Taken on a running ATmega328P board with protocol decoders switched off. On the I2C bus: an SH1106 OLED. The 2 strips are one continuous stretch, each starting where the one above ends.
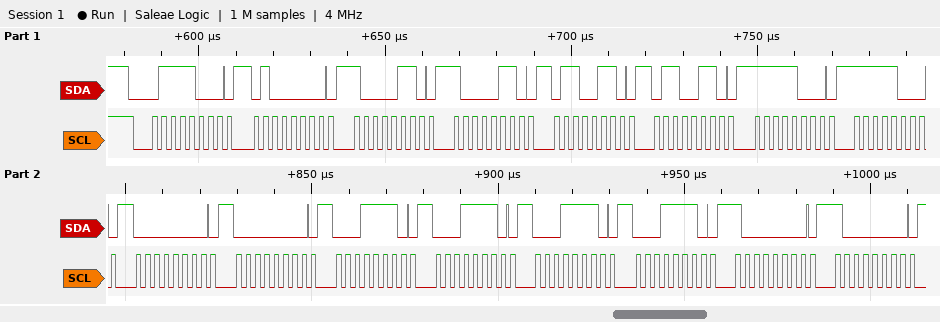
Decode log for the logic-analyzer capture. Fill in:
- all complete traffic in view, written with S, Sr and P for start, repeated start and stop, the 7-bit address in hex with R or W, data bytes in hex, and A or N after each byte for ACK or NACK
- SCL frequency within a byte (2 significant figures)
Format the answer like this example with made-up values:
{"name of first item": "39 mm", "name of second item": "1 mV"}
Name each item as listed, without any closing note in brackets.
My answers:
{"all complete traffic in view, written with S, Sr and P for start, repeated start and stop, the 7-bit address in hex with R or W, data bytes in hex, and A or N after each byte for ACK or NACK": "S 3CW A 40 A 86 A 86 A 66 A 66 A F8 A F8 A 00 A 00 A 1E A 1E A 1E A 1E A 80 A 80 A", "SCL frequency within a byte": "400 kHz"}
